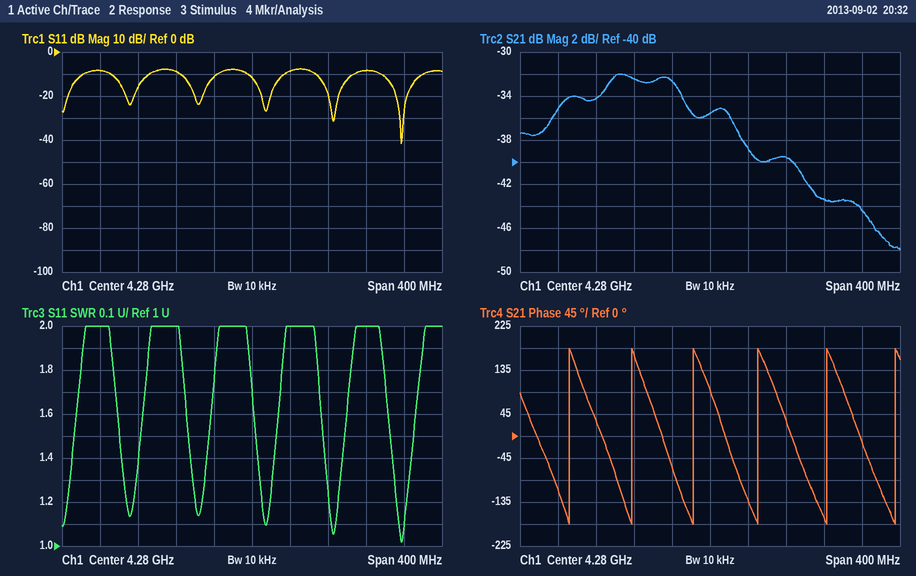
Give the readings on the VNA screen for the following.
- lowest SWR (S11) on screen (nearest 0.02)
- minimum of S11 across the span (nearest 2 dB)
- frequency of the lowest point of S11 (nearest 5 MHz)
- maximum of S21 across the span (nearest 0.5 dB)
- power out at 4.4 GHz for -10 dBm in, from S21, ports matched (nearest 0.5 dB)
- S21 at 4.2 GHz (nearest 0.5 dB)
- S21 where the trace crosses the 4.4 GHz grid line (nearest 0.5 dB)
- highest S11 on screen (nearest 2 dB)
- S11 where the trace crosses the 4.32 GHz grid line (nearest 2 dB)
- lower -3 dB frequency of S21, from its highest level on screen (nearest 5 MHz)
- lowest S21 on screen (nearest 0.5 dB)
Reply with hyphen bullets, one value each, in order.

- 1.02
- -42 dB
- 4.435 GHz
- -32.0 dB
- -53.5 dBm
- -32.5 dB
- -43.5 dB
- -8 dB
- -8 dB
- 4.120 GHz
- -48.0 dB
